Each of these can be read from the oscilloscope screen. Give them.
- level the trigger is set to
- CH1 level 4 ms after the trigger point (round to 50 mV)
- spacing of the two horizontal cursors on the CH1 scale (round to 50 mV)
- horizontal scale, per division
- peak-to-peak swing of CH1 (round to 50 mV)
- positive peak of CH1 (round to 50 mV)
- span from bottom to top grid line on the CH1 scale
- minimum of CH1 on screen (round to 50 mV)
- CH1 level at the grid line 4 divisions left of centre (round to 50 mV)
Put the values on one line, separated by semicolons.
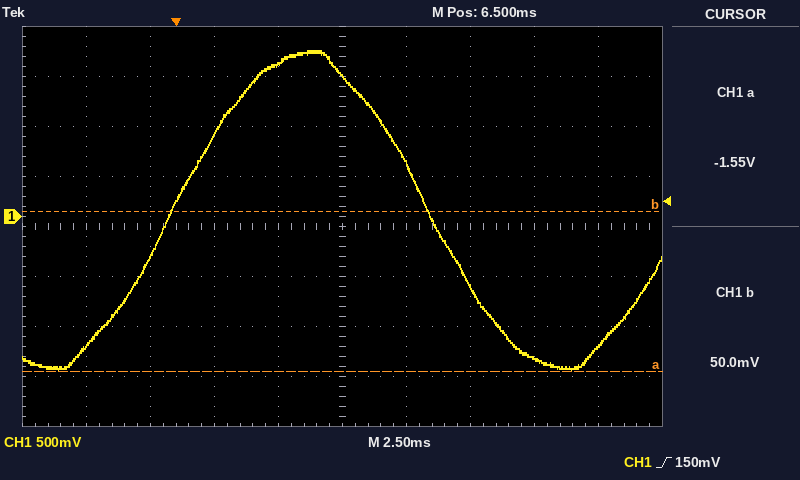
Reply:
150 mV; 1.50 V; 1.60 V; 2.5 ms; 3.20 V; 1.65 V; 4 V; -1.55 V; -1.30 V
